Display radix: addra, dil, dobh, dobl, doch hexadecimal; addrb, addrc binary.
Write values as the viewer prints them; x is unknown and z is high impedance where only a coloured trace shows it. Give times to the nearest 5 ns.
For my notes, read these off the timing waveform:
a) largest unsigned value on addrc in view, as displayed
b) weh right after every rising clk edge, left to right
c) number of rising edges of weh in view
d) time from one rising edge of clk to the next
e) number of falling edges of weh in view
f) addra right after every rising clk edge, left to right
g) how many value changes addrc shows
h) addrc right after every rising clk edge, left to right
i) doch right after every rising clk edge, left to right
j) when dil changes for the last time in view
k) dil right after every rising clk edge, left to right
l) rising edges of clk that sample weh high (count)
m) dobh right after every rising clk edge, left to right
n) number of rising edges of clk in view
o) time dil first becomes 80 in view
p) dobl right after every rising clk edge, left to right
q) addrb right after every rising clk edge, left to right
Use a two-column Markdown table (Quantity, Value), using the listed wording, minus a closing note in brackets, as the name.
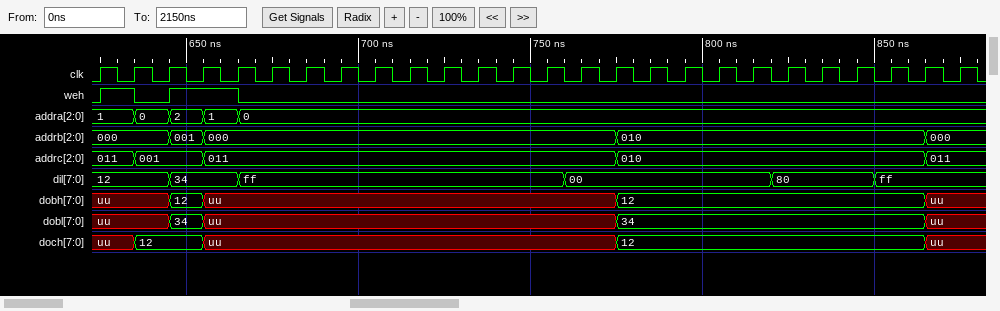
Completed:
| Quantity | Value |
|---|---|
| largest unsigned value on addrc in view, as displayed | 011 |
| weh right after every rising clk edge, left to right | 1 0 1 1 0 0 0 0 0 0 0 0 0 0 0 0 0 0 0 0 0 0 0 0 0 0 |
| number of rising edges of weh in view | 2 |
| time from one rising edge of clk to the next | 10 ns |
| number of falling edges of weh in view | 2 |
| addra right after every rising clk edge, left to right | 1, 0, 2, 1, 0, 0, 0, 0, 0, 0, 0, 0, 0, 0, 0, 0, 0, 0, 0, 0, 0, 0, 0, 0, 0, 0 |
| how many value changes addrc shows | 4 |
| addrc right after every rising clk edge, left to right | 011, 001, 001, 011, 011, 011, 011, 011, 011, 011, 011, 011, 011, 011, 011, 010, 010, 010, 010, 010, 010, 010, 010, 010, 011, 011 |
| doch right after every rising clk edge, left to right | uu, 12, 12, uu, uu, uu, uu, uu, uu, uu, uu, uu, uu, uu, uu, 12, 12, 12, 12, 12, 12, 12, 12, 12, uu, uu |
| when dil changes for the last time in view | 850 ns |
| dil right after every rising clk edge, left to right | 12, 12, 34, 34, ff, ff, ff, ff, ff, ff, ff, ff, ff, ff, 00, 00, 00, 00, 00, 00, 80, 80, 80, ff, ff, ff |
| rising edges of clk that sample weh high | 3 |
| dobh right after every rising clk edge, left to right | uu, uu, 12, uu, uu, uu, uu, uu, uu, uu, uu, uu, uu, uu, uu, 12, 12, 12, 12, 12, 12, 12, 12, 12, uu, uu |
| number of rising edges of clk in view | 26 |
| time dil first becomes 80 in view | 820 ns |
| dobl right after every rising clk edge, left to right | uu, uu, 34, uu, uu, uu, uu, uu, uu, uu, uu, uu, uu, uu, uu, 34, 34, 34, 34, 34, 34, 34, 34, 34, uu, uu |
| addrb right after every rising clk edge, left to right | 000, 000, 001, 000, 000, 000, 000, 000, 000, 000, 000, 000, 000, 000, 000, 010, 010, 010, 010, 010, 010, 010, 010, 010, 000, 000 |
